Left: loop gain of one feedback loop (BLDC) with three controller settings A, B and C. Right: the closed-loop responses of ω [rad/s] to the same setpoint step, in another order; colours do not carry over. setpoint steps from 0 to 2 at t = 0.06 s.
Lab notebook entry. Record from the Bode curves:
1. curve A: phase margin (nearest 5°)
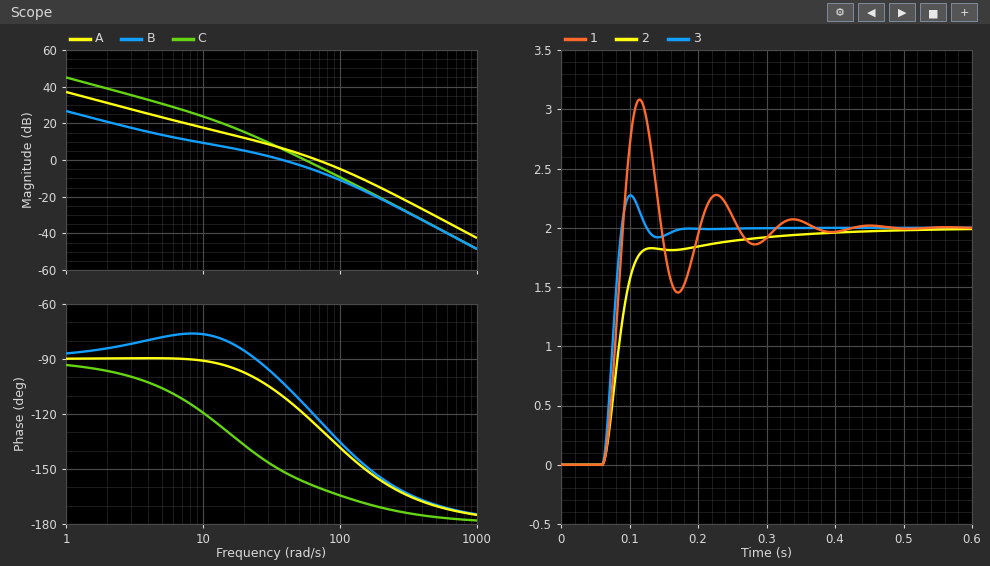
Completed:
55°
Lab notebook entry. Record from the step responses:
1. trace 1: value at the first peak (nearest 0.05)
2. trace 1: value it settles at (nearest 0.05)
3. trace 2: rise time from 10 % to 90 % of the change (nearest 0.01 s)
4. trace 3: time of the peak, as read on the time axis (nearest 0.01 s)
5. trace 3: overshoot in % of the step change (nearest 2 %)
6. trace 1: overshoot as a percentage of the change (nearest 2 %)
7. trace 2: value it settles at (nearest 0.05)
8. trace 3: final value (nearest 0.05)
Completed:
3.10
2.00
0.05 s
0.10 s
14 %
54 %
2.00
2.00
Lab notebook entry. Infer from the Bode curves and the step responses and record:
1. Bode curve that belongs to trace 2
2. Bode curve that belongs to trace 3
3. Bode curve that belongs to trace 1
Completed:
B
A
C
